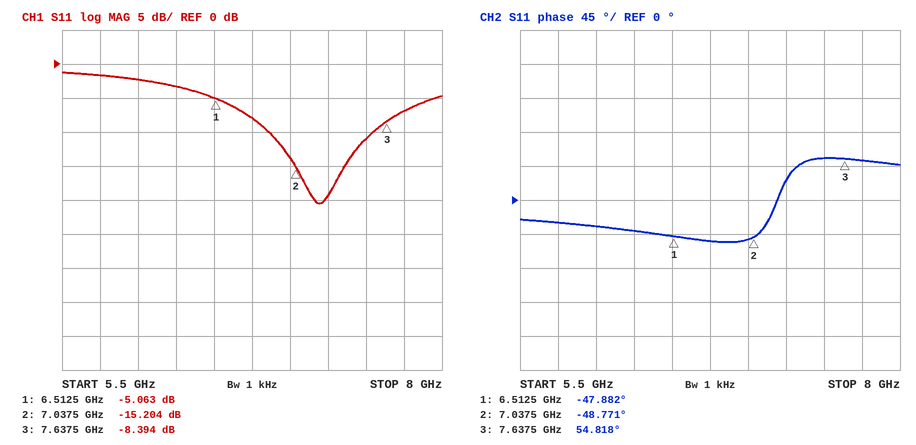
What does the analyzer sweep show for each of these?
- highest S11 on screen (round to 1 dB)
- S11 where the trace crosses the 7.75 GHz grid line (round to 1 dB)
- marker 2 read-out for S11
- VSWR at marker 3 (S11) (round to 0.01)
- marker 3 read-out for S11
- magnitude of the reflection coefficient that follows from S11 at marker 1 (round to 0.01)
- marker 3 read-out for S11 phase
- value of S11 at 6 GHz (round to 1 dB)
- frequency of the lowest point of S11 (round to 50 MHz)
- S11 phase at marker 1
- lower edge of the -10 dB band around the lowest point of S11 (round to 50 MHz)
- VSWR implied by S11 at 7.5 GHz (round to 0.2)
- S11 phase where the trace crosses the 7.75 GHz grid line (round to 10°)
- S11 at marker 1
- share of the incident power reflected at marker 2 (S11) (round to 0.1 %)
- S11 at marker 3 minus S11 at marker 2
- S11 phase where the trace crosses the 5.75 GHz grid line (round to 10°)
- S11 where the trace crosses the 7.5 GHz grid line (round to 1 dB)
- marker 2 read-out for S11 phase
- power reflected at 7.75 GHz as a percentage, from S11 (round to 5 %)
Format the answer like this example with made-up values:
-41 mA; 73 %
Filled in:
-1 dB; -7 dB; -15.204 dB; 2.23; -8.394 dB; 0.56; 54.818°; -2 dB; 7.20 GHz; -47.882°; 6.85 GHz; 1.8; 50°; -5.063 dB; 3.0 %; 6.810 dB; -30°; -11 dB; -48.771°; 20 %
